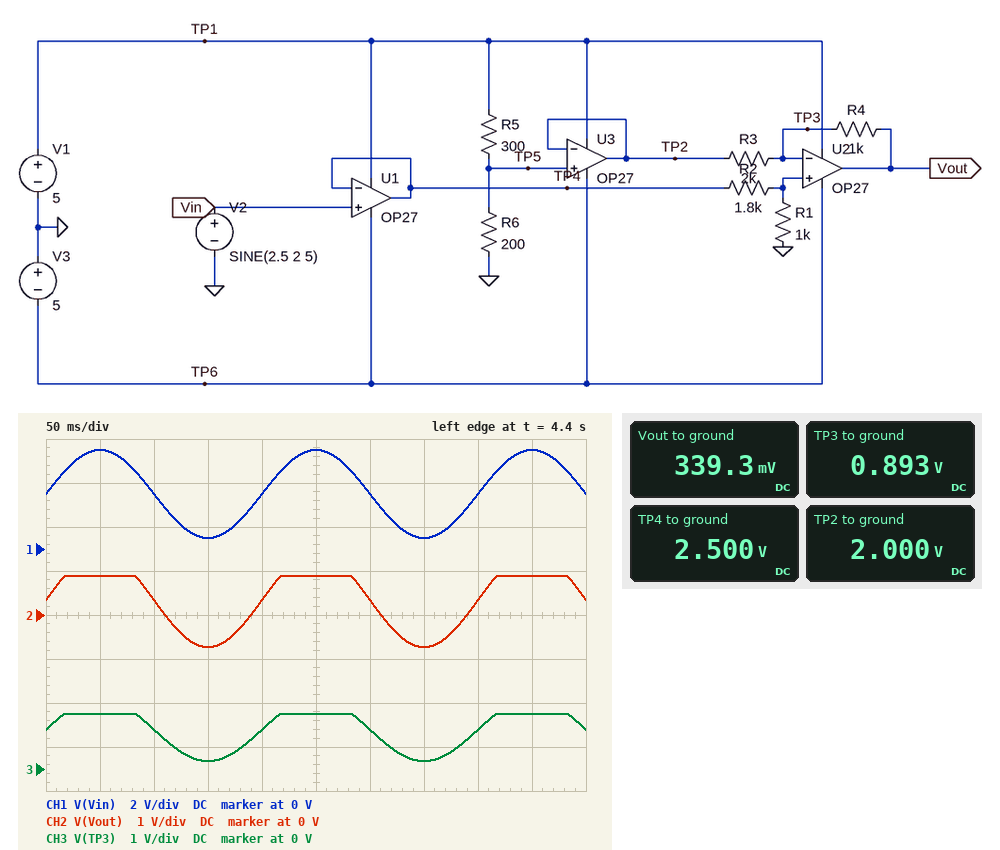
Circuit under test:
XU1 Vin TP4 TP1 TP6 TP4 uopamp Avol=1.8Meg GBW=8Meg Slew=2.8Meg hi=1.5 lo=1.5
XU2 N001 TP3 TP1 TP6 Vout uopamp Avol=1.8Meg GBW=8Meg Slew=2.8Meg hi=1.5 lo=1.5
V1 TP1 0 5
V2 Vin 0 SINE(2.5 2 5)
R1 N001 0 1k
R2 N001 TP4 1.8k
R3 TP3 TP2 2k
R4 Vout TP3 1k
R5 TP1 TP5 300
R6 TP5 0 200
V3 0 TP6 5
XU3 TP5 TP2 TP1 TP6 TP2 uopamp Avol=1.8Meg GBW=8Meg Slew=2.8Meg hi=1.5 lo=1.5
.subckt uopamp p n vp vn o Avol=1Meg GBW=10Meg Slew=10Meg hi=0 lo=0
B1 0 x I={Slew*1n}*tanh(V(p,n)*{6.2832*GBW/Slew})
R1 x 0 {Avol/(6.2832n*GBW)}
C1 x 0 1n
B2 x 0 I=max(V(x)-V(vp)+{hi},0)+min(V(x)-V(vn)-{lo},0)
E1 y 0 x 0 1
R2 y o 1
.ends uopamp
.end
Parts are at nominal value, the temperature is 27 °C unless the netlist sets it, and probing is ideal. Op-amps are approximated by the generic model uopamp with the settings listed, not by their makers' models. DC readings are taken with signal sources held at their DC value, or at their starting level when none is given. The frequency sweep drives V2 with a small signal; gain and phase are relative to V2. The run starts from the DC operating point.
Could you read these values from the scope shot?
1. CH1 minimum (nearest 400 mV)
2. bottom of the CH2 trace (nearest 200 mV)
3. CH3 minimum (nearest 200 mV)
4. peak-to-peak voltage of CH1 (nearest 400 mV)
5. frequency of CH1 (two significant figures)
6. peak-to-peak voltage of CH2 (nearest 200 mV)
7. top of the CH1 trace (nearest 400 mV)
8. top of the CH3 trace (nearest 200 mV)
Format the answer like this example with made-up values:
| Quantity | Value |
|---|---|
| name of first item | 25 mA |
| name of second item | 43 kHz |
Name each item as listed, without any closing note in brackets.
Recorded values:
| Quantity | Value |
|---|---|
| CH1 minimum | 400 mV |
| bottom of the CH2 trace | -800 mV |
| CH3 minimum | 200 mV |
| peak-to-peak voltage of CH1 | 4.0 V |
| frequency of CH1 | 5.0 Hz |
| peak-to-peak voltage of CH2 | 1.6 V |
| top of the CH1 trace | 4.4 V |
| top of the CH3 trace | 1.2 V |
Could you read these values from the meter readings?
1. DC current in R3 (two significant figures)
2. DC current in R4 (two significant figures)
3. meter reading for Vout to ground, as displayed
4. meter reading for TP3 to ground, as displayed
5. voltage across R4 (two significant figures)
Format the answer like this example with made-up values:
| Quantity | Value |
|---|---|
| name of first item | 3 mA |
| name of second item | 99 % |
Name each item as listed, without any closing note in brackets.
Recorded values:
| Quantity | Value |
|---|---|
| DC current in R3 | 550 µA |
| DC current in R4 | 550 µA |
| meter reading for Vout to ground, as displayed | 339.3 mV |
| meter reading for TP3 to ground, as displayed | 0.893 V |
| voltage across R4 | 550 mV |
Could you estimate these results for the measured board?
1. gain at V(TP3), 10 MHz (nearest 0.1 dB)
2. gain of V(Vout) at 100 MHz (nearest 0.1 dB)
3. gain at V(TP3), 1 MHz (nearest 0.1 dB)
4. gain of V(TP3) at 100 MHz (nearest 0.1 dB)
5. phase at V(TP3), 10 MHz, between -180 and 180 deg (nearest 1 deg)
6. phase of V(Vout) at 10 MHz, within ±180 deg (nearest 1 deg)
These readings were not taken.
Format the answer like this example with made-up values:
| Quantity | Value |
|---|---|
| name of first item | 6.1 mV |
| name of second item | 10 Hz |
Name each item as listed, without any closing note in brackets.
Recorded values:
| Quantity | Value |
|---|---|
| gain at V(TP3), 10 MHz | -19.6 dB |
| gain of V(Vout) at 100 MHz | -52.9 dB |
| gain at V(TP3), 1 MHz | -9.2 dB |
| gain of V(TP3) at 100 MHz | -56.4 dB |
| phase at V(TP3), 10 MHz, between -180 and 180 deg | -113 deg |
| phase of V(Vout) at 10 MHz, within ±180 deg | -113 deg |
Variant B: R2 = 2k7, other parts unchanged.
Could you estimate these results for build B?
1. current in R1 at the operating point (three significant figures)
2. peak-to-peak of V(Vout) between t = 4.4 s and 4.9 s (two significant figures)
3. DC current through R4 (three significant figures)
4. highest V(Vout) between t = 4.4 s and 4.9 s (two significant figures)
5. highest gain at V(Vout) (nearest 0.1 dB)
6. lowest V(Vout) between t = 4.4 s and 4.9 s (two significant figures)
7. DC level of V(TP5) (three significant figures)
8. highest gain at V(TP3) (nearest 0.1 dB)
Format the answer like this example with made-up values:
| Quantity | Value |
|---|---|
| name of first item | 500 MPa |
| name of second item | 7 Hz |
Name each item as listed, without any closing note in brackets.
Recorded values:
| Quantity | Value |
|---|---|
| current in R1 at the operating point | 676 µA |
| peak-to-peak of V(Vout) between t = 4.4 s and 4.9 s | 1.2 V |
| DC current through R4 | 662 µA |
| highest V(Vout) between t = 4.4 s and 4.9 s | 420 mV |
| highest gain at V(Vout) | -7.8 dB |
| lowest V(Vout) between t = 4.4 s and 4.9 s | -800 mV |
| DC level of V(TP5) | 2.00 V |
| highest gain at V(TP3) | -11.4 dB |
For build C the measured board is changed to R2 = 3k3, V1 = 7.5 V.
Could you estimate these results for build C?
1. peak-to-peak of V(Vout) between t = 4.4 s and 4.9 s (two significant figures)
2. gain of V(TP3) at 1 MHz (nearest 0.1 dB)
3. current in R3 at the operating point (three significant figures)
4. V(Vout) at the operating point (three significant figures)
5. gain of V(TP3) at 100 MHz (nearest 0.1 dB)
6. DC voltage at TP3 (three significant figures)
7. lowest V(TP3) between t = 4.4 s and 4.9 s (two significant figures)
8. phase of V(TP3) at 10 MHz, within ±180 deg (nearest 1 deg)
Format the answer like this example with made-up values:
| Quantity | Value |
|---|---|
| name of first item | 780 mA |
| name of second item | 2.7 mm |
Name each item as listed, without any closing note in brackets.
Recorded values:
| Quantity | Value |
|---|---|
| peak-to-peak of V(Vout) between t = 4.4 s and 4.9 s | 1.4 V |
| gain of V(TP3) at 1 MHz | -12.9 dB |
| current in R3 at the operating point | 1.21 mA |
| V(Vout) at the operating point | -628 mV |
| gain of V(TP3) at 100 MHz | -60.1 dB |
| DC voltage at TP3 | 581 mV |
| lowest V(TP3) between t = 4.4 s and 4.9 s | 120 mV |
| phase of V(TP3) at 10 MHz, within ±180 deg | -113 deg |
